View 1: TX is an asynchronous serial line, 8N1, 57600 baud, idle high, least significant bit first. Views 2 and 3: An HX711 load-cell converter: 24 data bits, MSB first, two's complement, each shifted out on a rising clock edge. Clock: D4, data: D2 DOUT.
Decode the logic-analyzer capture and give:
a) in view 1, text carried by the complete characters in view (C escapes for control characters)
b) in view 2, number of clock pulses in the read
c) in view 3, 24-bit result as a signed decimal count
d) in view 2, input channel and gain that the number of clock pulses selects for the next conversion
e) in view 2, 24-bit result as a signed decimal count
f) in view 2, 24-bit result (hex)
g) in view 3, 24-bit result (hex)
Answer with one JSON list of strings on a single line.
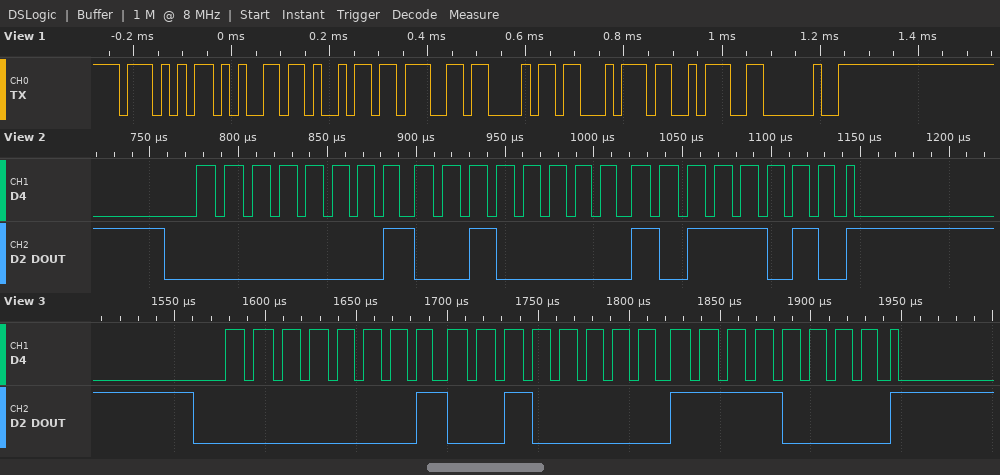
["\"Weight: \"", "25", "73968", "channel A, gain 128", "73914", "0x0120BA", "0x0120F0"]
